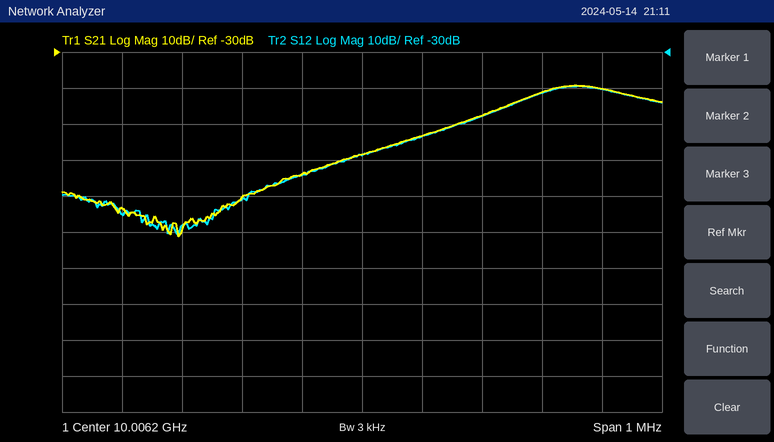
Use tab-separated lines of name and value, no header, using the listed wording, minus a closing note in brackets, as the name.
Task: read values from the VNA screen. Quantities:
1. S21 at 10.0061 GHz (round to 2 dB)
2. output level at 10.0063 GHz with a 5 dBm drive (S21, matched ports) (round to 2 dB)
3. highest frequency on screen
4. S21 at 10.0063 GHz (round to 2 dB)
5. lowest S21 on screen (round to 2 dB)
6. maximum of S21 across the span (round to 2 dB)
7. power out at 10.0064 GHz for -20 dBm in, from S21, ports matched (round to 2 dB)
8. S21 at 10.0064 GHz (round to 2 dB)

S21 at 10.0061 GHz	-64 dB
output level at 10.0063 GHz with a 5 dBm drive (S21, matched ports)	-48 dBm
highest frequency on screen	10.0067 GHz
S21 at 10.0063 GHz	-54 dB
lowest S21 on screen	-82 dB
maximum of S21 across the span	-40 dB
power out at 10.0064 GHz for -20 dBm in, from S21, ports matched	-68 dBm
S21 at 10.0064 GHz	-48 dB
